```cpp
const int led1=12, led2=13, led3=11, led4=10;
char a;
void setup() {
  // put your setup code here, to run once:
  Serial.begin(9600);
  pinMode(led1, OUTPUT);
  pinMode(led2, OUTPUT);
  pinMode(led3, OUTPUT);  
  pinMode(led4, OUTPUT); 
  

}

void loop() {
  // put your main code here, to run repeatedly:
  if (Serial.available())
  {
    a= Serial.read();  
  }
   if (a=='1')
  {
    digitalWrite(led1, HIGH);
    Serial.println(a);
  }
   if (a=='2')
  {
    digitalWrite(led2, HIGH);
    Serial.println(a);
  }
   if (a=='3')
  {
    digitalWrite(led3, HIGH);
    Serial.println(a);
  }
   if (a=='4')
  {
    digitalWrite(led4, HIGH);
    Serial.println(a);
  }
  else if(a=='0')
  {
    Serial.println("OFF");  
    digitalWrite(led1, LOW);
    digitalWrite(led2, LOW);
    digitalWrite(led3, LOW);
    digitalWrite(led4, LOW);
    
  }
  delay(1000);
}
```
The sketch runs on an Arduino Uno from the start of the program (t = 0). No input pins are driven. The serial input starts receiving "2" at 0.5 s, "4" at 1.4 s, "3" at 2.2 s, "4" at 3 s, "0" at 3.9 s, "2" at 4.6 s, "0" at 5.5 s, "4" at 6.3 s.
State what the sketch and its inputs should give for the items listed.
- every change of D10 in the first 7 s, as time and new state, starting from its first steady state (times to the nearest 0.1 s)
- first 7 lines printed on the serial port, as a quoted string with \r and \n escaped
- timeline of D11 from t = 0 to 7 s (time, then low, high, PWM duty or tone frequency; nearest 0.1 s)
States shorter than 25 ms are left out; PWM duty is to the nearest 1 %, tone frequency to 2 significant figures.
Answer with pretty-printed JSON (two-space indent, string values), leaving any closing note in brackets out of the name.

{
  "every change of D10 in the first 7 s, as time and new state, starting from its first steady state": "0 s low; 2 s high; 5 s low",
  "first 7 lines printed on the serial port, as a quoted string with \\r and \\n escaped": "\"2\\r\\n4\\r\\n3\\r\\n4\\r\\nOFF\\r\\n2\\r\\nOFF\\r\\n\"",
  "timeline of D11 from t = 0 to 7 s": "0 s low; 3 s high; 5 s low"
}
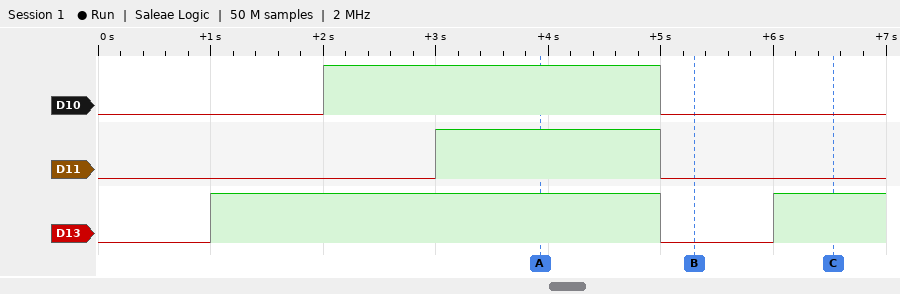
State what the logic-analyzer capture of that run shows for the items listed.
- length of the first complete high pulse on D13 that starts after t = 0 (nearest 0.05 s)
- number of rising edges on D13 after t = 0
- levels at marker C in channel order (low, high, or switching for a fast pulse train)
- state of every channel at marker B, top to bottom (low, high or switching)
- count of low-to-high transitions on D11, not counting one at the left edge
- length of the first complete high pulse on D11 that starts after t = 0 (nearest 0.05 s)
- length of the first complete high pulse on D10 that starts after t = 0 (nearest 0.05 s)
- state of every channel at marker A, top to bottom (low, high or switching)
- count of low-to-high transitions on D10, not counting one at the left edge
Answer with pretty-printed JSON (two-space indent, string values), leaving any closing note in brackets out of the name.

{
  "length of the first complete high pulse on D13 that starts after t = 0": "4.00 s",
  "number of rising edges on D13 after t = 0": "2",
  "levels at marker C in channel order": "D10 low, D11 low, D13 high",
  "state of every channel at marker B, top to bottom": "D10 low, D11 low, D13 low",
  "count of low-to-high transitions on D11, not counting one at the left edge": "1",
  "length of the first complete high pulse on D11 that starts after t = 0": "2.00 s",
  "length of the first complete high pulse on D10 that starts after t = 0": "3.00 s",
  "state of every channel at marker A, top to bottom": "D10 high, D11 high, D13 high",
  "count of low-to-high transitions on D10, not counting one at the left edge": "1"
}
